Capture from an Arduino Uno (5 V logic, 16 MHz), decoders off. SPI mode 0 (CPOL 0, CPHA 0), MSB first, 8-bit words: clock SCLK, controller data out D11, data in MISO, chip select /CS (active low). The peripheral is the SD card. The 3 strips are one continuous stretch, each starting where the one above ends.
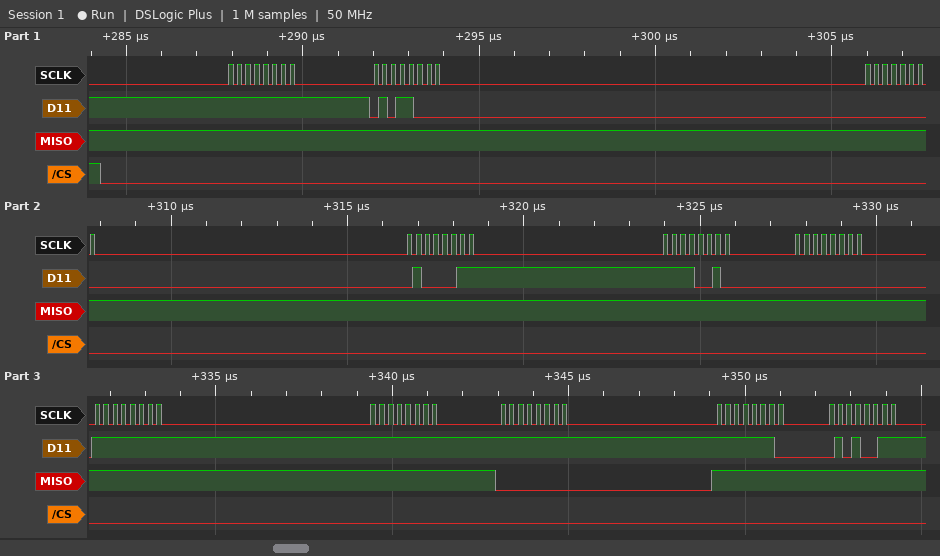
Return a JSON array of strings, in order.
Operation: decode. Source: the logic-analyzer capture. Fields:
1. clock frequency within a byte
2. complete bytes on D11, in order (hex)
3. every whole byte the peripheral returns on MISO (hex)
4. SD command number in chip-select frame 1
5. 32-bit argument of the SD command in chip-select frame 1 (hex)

["4 MHz", "FF 58 00 43 F2 00 FF FF FF FE 53", "FF FF FF FF FF FF FF FF 00 FF FF", "CMD24", "0x0043F200"]
